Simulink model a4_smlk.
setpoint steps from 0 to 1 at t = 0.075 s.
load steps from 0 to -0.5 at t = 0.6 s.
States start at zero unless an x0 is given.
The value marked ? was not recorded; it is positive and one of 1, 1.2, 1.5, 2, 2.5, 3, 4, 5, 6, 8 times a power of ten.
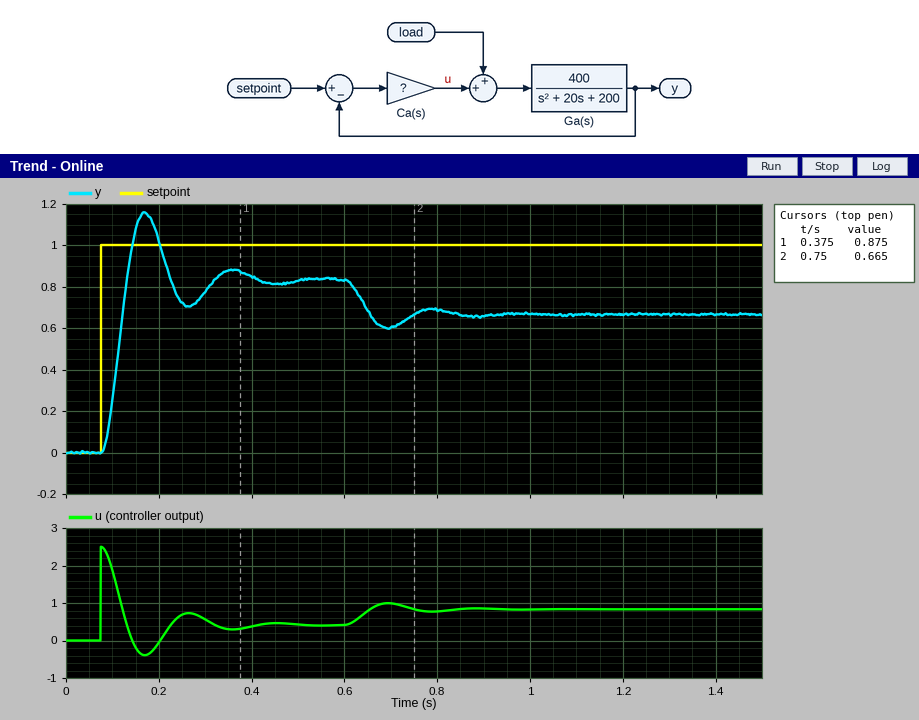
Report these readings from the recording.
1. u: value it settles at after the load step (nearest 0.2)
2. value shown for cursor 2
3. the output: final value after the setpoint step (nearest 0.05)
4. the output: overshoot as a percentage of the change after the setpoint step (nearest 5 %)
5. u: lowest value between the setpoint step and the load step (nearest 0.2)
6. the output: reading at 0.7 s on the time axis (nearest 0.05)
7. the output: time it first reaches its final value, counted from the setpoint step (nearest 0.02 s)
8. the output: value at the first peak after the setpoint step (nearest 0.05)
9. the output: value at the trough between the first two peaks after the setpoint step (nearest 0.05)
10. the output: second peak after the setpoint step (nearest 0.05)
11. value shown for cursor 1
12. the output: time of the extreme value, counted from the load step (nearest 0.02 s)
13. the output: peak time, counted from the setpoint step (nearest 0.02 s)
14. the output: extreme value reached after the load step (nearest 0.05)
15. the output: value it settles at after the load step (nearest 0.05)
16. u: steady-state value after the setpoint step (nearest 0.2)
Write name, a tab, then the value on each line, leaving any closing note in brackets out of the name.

u: value it settles at after the load step	0.8
value shown for cursor 2	0.665
the output: final value after the setpoint step	0.85
the output: overshoot as a percentage of the change after the setpoint step	40 %
u: lowest value between the setpoint step and the load step	-0.4
the output: reading at 0.7 s on the time axis	0.60
the output: time it first reaches its final value, counted from the setpoint step	0.06 s
the output: value at the first peak after the setpoint step	1.15
the output: value at the trough between the first two peaks after the setpoint step	0.70
the output: second peak after the setpoint step	0.90
value shown for cursor 1	0.875
the output: time of the extreme value, counted from the load step	0.10 s
the output: peak time, counted from the setpoint step	0.10 s
the output: extreme value reached after the load step	0.60
the output: value it settles at after the load step	0.65
u: steady-state value after the setpoint step	0.4
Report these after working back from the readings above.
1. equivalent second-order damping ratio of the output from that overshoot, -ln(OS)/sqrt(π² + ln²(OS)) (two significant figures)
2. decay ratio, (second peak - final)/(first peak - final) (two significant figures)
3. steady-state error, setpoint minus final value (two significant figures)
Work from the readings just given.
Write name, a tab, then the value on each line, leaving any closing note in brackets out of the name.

equivalent second-order damping ratio of the output from that overshoot, -ln(OS)/sqrt(π² + ln²(OS))	0.28
decay ratio, (second peak - final)/(first peak - final)	0.17
steady-state error, setpoint minus final value	0.15
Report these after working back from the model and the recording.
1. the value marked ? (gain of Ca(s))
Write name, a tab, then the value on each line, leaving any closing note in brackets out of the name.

the value marked ? (gain of Ca(s))	2.5
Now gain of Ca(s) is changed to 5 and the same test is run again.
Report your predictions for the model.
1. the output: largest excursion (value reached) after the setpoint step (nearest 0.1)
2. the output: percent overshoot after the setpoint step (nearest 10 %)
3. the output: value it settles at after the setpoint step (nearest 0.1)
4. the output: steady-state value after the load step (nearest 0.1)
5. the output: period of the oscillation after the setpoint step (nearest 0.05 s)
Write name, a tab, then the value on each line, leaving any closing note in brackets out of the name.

the output: largest excursion (value reached) after the setpoint step	1.4
the output: percent overshoot after the setpoint step	50 %
the output: value it settles at after the setpoint step	0.9
the output: steady-state value after the load step	0.8
the output: period of the oscillation after the setpoint step	0.15 s
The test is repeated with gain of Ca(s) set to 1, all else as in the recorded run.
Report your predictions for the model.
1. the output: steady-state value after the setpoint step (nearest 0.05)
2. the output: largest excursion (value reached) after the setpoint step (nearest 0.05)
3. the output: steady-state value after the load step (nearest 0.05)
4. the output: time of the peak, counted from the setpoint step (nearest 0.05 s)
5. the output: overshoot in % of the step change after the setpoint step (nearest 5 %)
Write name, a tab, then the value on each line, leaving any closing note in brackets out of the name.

the output: steady-state value after the setpoint step	0.65
the output: largest excursion (value reached) after the setpoint step	0.85
the output: steady-state value after the load step	0.35
the output: time of the peak, counted from the setpoint step	0.15 s
the output: overshoot in % of the step change after the setpoint step	25 %
